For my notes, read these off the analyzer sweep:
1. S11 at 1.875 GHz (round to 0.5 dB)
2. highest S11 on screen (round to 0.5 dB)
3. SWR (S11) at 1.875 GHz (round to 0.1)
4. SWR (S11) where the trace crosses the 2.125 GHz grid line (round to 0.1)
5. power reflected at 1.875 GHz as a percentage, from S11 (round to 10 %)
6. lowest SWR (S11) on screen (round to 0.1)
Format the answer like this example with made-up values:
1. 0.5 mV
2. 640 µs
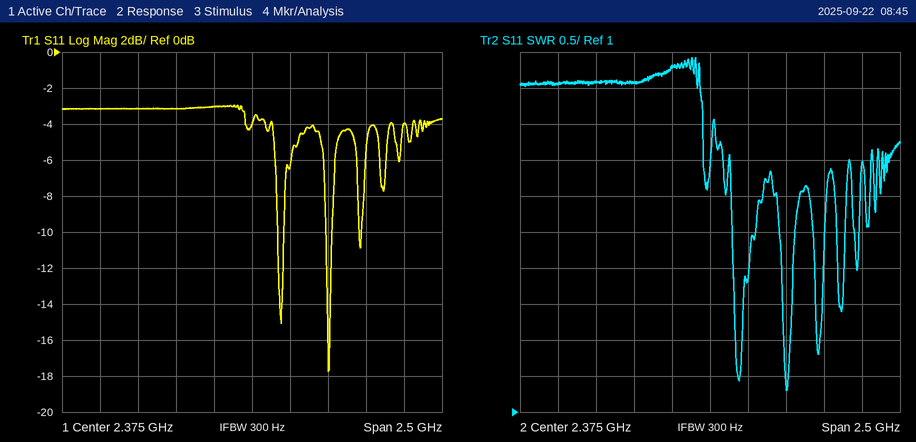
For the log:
1. -3.0 dB
2. -3.0 dB
3. 5.6
4. 5.8
5. 50 %
6. 1.3
